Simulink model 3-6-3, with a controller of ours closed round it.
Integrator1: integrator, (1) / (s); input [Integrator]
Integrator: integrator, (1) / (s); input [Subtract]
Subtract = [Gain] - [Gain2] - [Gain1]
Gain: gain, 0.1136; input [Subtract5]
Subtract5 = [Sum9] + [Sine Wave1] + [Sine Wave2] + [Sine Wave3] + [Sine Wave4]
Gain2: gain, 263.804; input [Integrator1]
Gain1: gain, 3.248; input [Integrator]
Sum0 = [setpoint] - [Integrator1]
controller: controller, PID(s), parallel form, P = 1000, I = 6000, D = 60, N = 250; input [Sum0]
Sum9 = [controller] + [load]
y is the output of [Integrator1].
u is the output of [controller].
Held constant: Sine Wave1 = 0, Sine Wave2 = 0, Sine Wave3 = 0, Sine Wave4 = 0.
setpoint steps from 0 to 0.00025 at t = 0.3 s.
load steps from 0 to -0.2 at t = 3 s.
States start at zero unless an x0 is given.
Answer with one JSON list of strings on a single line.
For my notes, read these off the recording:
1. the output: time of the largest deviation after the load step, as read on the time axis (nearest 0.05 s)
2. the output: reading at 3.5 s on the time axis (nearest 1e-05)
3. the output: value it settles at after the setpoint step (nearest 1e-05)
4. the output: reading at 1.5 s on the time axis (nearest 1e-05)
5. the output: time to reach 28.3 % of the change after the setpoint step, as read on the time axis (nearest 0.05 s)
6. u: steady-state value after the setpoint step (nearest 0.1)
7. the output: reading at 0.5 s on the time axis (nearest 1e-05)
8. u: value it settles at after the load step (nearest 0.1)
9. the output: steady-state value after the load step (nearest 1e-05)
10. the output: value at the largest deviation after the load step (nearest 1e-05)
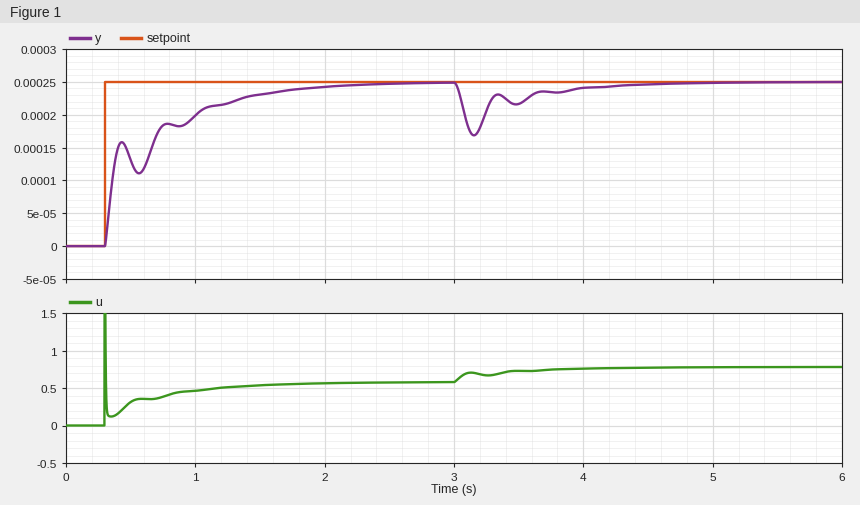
["3.15 s", "0.00022", "0.00025", "0.00023", "0.35 s", "0.6", "0.00013", "0.8", "0.00025", "0.00017"]
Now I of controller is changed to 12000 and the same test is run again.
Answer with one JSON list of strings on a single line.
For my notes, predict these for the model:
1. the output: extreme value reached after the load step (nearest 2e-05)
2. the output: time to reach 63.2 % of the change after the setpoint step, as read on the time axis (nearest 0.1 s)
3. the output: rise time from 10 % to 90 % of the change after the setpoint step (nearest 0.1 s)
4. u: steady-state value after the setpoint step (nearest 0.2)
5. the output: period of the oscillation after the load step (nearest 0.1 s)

["0.00018", "0.4 s", "0.4 s", "0.6", "0.3 s"]
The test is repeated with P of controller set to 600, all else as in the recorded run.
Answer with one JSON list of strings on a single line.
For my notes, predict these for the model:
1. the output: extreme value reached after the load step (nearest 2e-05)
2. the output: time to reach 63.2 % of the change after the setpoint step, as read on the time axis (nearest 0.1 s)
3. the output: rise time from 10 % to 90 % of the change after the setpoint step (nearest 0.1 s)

["0.00016", "0.7 s", "1.0 s"]
